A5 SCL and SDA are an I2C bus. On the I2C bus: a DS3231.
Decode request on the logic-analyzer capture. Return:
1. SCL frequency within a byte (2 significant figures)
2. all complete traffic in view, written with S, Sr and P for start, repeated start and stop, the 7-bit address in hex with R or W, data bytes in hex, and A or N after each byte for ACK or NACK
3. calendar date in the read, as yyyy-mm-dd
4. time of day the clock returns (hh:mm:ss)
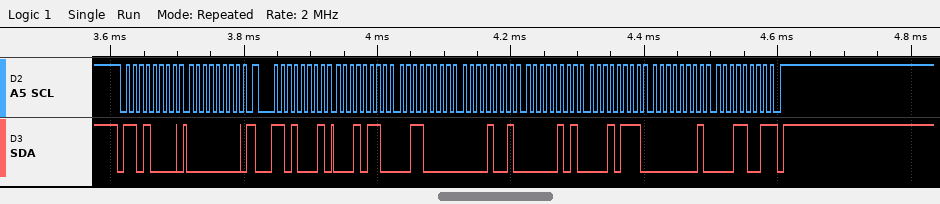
100 kHz
S 68W A 00 A Sr 68R A 16 A 30 A 09 A 05 A 17 A 01 A 19 N P
2019-01-17
09:30:16
